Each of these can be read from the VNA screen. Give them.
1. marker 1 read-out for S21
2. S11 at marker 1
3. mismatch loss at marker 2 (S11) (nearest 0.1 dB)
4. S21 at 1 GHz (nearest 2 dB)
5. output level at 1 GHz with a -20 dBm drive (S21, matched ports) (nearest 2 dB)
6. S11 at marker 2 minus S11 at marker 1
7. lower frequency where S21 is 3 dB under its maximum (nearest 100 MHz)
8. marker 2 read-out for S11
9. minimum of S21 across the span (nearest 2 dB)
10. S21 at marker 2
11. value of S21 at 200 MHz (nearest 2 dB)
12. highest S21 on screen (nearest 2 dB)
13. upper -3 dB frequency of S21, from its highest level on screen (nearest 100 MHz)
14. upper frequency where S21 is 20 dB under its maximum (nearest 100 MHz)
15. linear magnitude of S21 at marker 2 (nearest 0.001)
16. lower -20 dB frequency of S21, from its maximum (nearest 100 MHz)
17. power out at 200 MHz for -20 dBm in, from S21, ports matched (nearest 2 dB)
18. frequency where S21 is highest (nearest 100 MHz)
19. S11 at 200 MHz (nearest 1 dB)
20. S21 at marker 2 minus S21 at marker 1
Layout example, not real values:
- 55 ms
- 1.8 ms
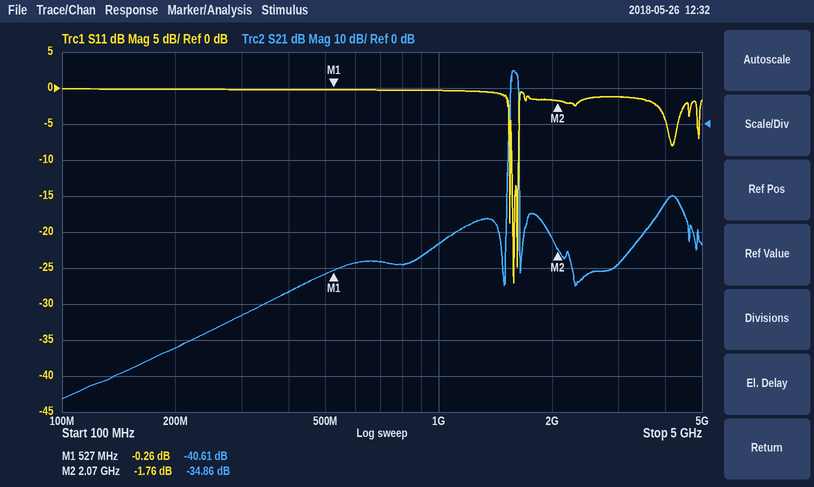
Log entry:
- -40.61 dB
- -0.26 dB
- 4.8 dB
- -34 dB
- -54 dBm
- -1.50 dB
- 1.6 GHz
- -1.76 dB
- -76 dB
- -34.86 dB
- -62 dB
- 14 dB
- 1.6 GHz
- 1.6 GHz
- 0.018
- 1.5 GHz
- -82 dBm
- 1.6 GHz
- 0 dB
- 5.75 dB
